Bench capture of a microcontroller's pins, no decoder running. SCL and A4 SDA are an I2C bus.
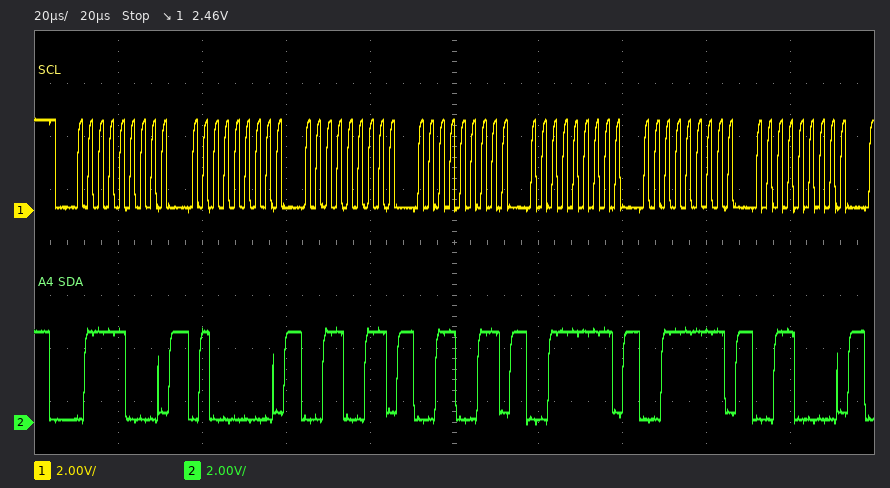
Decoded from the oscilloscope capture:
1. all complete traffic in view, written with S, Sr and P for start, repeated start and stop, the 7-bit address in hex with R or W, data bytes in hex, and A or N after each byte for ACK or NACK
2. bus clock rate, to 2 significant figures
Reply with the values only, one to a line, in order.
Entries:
S 3CW A 40 A 33 A 33 A 3F A 3F A 30 A
400 kHz
